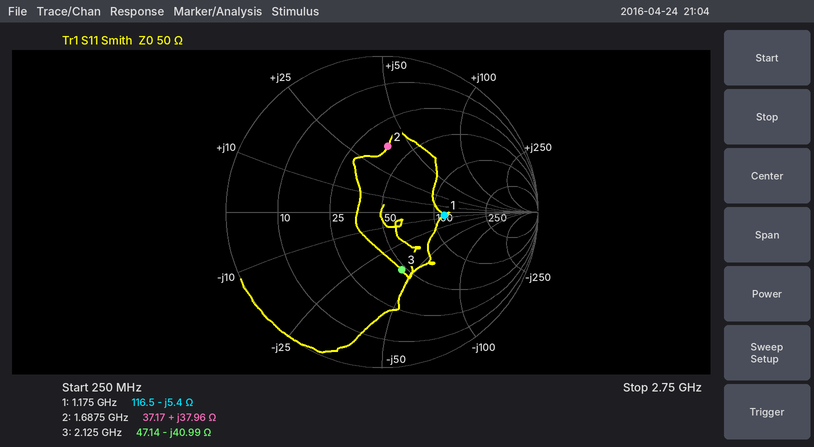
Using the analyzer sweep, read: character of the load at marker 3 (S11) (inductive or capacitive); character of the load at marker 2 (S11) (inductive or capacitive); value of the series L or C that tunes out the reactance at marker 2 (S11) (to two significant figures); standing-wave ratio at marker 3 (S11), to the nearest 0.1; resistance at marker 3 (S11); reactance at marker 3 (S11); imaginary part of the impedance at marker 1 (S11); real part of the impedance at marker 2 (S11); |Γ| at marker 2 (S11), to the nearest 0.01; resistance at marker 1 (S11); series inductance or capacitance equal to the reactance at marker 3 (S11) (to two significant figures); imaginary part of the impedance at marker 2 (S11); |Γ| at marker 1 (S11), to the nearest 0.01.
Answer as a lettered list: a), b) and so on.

a) capacitive
b) inductive
c) 2.5 pF
d) 2.3
e) 47.14 Ω
f) -40.99 Ω
g) -5.4 Ω
h) 37.17 Ω
i) 0.42
j) 116.5 Ω
k) 1.8 pF
l) +37.96 Ω
m) 0.40
